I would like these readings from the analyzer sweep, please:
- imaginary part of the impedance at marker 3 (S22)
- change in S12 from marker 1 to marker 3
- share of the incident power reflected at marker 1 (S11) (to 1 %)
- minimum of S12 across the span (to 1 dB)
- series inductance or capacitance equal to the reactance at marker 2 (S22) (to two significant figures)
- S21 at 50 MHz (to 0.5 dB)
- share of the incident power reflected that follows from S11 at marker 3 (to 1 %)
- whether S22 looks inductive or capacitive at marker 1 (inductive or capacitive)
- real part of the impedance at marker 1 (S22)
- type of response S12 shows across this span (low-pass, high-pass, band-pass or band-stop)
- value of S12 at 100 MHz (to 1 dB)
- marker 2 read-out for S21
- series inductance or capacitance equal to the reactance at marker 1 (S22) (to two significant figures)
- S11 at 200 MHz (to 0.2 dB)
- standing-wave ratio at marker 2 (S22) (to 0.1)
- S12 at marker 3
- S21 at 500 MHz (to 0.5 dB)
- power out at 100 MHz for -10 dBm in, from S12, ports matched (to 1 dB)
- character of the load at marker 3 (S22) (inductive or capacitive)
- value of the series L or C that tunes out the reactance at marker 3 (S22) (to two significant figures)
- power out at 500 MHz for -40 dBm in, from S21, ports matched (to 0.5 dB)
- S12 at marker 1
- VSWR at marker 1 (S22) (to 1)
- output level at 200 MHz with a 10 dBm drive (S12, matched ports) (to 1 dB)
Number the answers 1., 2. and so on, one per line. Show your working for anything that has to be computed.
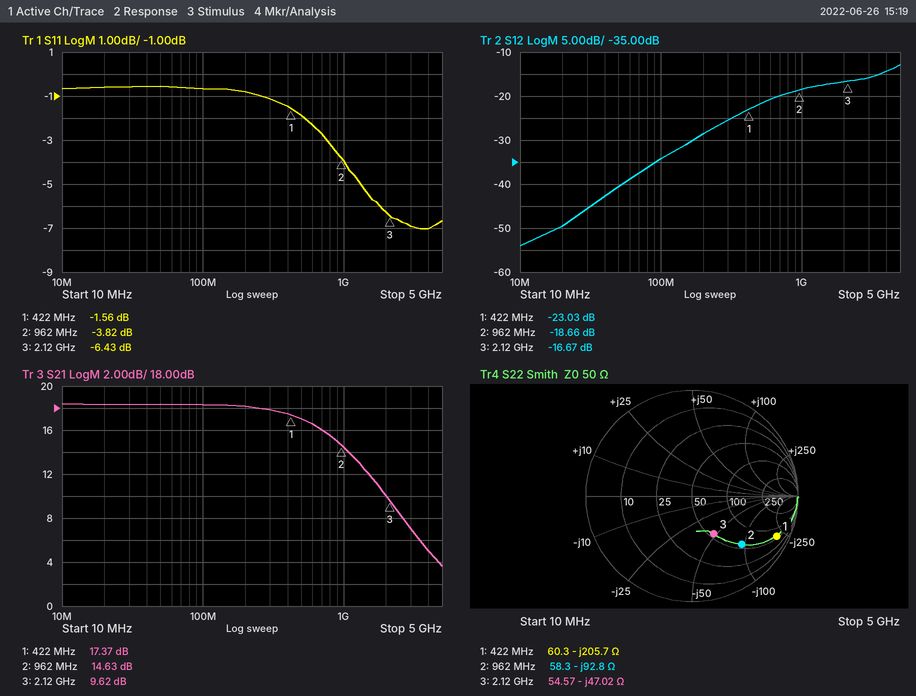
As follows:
1. -47.02 Ω
2. -16.67 − (-23.03) = 6.36 dB
3. 10^(-1.56/10) ≈ 70 %
4. -54 dB
5. C = 1/(2π × 962 MHz × 92.8 Ω) ≈ 1.8 pF
6. 18.5 dB
7. 10^(-6.43/10) ≈ 23 %
8. capacitive
9. 60.3 Ω
10. high-pass
11. -34 dB
12. 14.63 dB
13. C = 1/(2π × 422 MHz × 205.7 Ω) ≈ 1.8 pF
14. -0.8 dB
15. 4.8
16. -16.67 dB
17. 17.0 dB
18. -10 dBm + (-34 dB) = -44 dBm
19. capacitive
20. L = 47.02 Ω/(2π × 2.12 GHz) ≈ 3.5 nH
21. -40 dBm + (17.0 dB) = -23.0 dBm
22. -23.03 dB
23. 16
24. 10 dBm + (-29 dB) = -19 dBm
